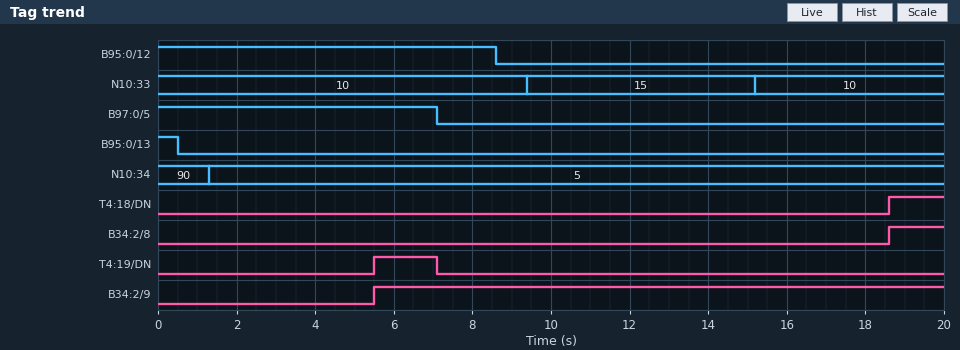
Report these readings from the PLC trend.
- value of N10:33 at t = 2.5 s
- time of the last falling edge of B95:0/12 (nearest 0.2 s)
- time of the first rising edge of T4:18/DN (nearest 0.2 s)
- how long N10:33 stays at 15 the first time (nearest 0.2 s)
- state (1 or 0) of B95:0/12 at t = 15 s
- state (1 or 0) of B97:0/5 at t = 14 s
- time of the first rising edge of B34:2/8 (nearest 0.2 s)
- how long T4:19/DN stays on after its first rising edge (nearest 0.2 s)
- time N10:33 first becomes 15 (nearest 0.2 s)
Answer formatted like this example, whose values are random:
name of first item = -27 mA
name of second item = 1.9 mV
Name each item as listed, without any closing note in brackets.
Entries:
value of N10:33 at t = 2.5 s = 10
time of the last falling edge of B95:0/12 = 8.6 s
time of the first rising edge of T4:18/DN = 18.6 s
how long N10:33 stays at 15 the first time = 5.8 s
state (1 or 0) of B95:0/12 at t = 15 s = 0
state (1 or 0) of B97:0/5 at t = 14 s = 0
time of the first rising edge of B34:2/8 = 18.6 s
how long T4:19/DN stays on after its first rising edge = 1.6 s
time N10:33 first becomes 15 = 9.4 s
